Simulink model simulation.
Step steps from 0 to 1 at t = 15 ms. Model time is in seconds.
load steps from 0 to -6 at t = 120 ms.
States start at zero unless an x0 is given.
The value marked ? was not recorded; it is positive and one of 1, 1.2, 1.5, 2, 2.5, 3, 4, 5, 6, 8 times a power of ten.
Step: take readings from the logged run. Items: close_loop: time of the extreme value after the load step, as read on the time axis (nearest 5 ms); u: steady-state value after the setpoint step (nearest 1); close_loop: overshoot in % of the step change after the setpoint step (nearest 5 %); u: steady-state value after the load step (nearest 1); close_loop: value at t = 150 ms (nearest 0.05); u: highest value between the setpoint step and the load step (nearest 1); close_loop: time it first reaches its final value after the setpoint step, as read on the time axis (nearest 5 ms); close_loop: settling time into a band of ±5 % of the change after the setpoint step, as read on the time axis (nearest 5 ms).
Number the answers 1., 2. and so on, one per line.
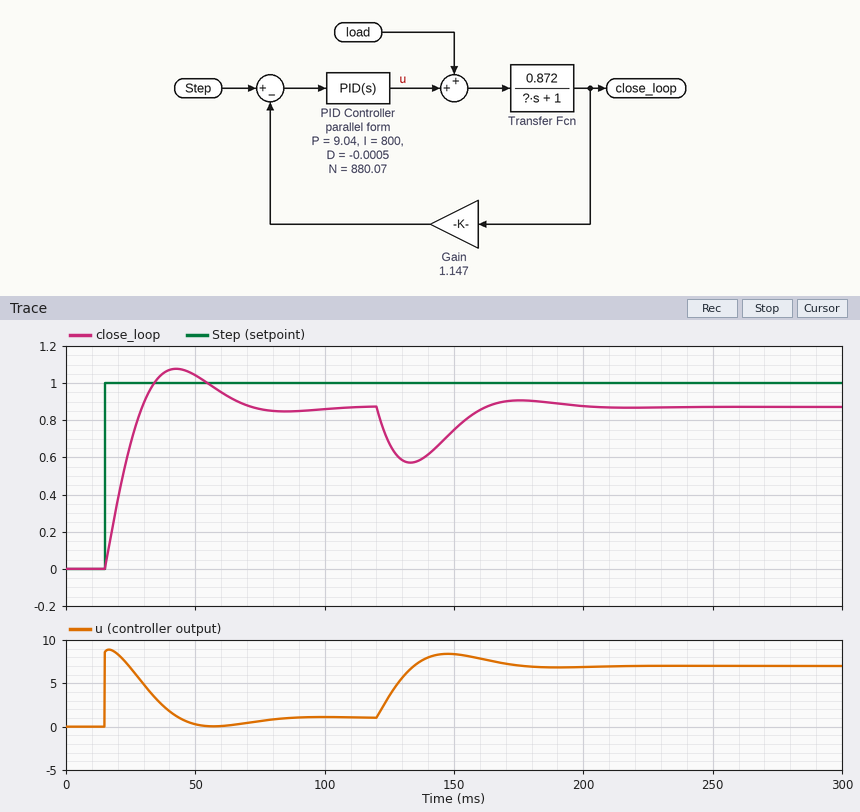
1. 135 ms
2. 1
3. 25 %
4. 7
5. 0.75
6. 9
7. 30 ms
8. 65 ms
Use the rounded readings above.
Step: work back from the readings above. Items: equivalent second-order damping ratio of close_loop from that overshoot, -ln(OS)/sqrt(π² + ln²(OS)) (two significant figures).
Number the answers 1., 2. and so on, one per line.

1. 0.40
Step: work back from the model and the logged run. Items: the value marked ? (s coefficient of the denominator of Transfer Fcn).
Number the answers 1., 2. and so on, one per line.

1. 0.1
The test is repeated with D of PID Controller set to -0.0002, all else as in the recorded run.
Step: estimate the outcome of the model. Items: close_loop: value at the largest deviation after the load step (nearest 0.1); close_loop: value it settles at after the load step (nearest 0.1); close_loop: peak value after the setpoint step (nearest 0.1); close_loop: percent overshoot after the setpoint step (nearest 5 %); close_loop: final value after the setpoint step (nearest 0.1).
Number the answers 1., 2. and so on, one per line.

1. 0.6
2. 0.9
3. 1.1
4. 25 %
5. 0.9
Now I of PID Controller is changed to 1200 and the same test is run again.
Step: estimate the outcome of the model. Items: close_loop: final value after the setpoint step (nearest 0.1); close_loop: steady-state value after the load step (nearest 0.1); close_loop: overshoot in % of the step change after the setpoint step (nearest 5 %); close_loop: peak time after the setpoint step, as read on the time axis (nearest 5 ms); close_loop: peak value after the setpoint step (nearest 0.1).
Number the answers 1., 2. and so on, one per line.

1. 0.9
2. 0.9
3. 30 %
4. 40 ms
5. 1.1
